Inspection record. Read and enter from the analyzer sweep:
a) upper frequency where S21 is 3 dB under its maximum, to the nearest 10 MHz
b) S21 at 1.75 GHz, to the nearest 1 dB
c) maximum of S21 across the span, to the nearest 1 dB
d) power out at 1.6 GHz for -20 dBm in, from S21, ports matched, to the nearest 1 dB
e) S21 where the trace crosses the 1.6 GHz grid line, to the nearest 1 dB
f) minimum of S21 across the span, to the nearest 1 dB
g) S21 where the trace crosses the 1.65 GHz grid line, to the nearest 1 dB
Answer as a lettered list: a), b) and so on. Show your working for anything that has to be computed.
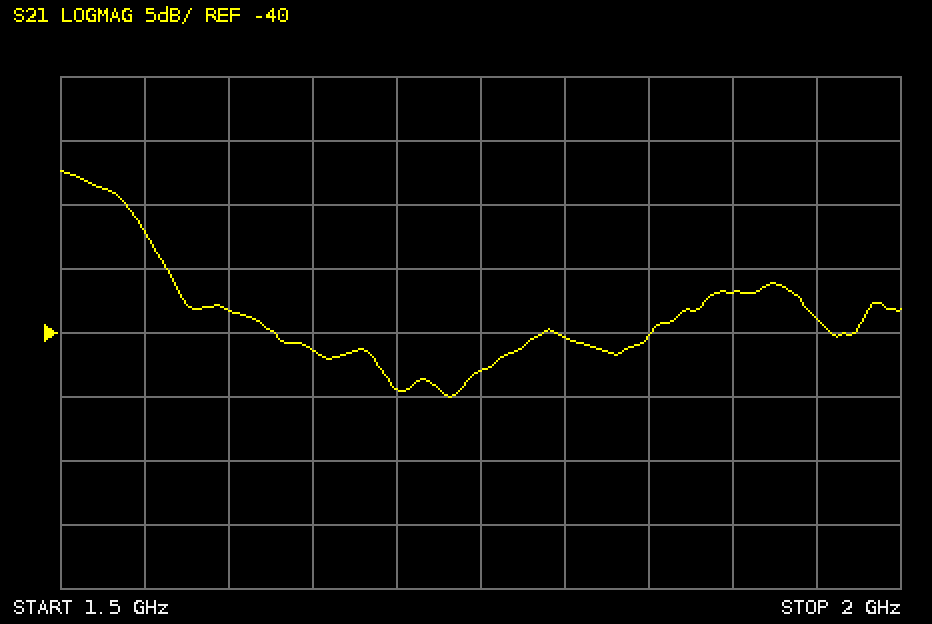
a) 1.54 GHz
b) -43 dB
c) -27 dB
d) -20 dBm + (-38 dB) = -58 dBm
e) -38 dB
f) -45 dB
g) -41 dB
